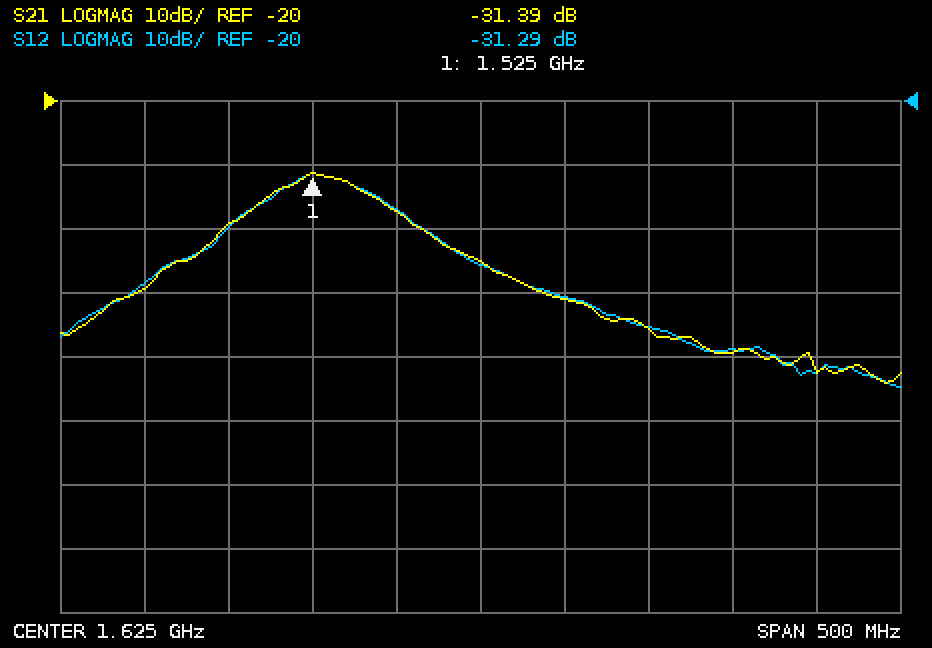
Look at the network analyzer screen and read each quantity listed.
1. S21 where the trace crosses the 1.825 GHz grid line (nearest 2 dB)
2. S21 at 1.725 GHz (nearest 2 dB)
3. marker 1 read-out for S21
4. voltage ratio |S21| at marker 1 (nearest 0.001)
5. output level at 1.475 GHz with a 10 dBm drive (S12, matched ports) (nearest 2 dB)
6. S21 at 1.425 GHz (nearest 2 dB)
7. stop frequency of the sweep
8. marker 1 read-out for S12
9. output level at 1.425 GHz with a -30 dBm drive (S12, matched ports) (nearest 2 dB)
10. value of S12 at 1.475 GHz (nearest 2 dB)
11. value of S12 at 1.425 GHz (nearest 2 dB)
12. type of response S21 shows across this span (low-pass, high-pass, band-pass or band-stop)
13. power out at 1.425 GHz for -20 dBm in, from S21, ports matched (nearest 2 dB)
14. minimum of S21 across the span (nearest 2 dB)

-62 dB
-56 dB
-31.39 dB
0.027
-30 dBm
-50 dB
1.875 GHz
-31.29 dB
-78 dBm
-40 dB
-48 dB
band-pass
-70 dBm
-64 dB
